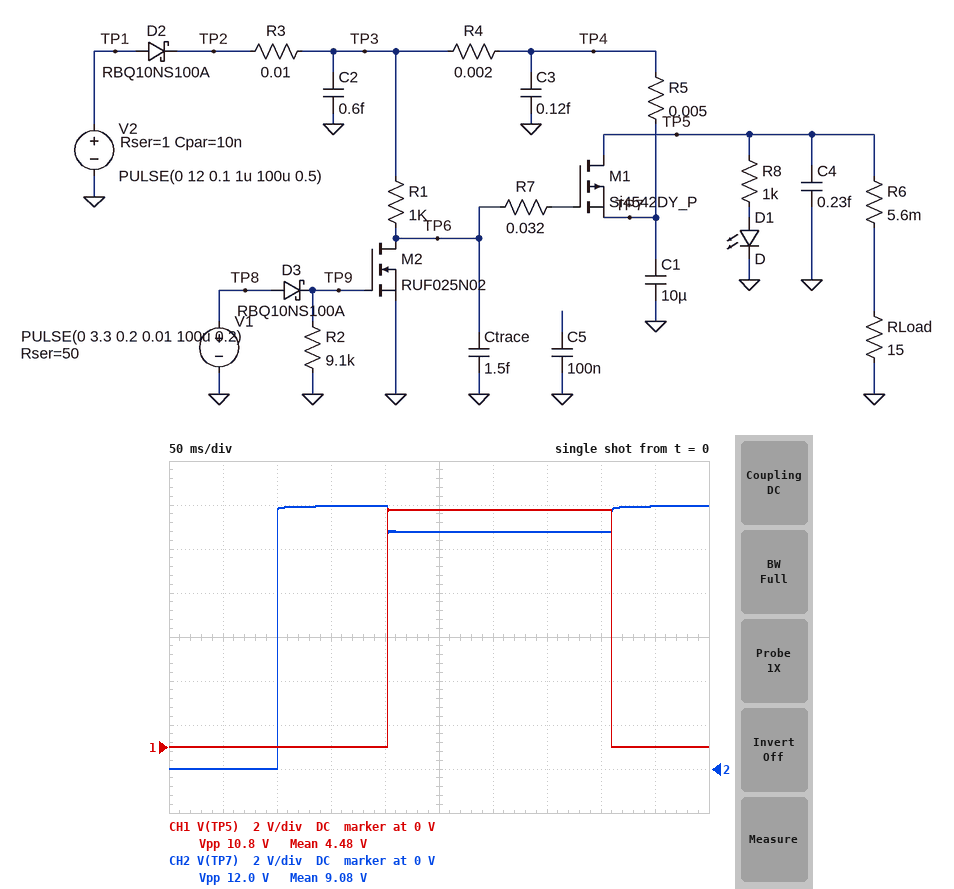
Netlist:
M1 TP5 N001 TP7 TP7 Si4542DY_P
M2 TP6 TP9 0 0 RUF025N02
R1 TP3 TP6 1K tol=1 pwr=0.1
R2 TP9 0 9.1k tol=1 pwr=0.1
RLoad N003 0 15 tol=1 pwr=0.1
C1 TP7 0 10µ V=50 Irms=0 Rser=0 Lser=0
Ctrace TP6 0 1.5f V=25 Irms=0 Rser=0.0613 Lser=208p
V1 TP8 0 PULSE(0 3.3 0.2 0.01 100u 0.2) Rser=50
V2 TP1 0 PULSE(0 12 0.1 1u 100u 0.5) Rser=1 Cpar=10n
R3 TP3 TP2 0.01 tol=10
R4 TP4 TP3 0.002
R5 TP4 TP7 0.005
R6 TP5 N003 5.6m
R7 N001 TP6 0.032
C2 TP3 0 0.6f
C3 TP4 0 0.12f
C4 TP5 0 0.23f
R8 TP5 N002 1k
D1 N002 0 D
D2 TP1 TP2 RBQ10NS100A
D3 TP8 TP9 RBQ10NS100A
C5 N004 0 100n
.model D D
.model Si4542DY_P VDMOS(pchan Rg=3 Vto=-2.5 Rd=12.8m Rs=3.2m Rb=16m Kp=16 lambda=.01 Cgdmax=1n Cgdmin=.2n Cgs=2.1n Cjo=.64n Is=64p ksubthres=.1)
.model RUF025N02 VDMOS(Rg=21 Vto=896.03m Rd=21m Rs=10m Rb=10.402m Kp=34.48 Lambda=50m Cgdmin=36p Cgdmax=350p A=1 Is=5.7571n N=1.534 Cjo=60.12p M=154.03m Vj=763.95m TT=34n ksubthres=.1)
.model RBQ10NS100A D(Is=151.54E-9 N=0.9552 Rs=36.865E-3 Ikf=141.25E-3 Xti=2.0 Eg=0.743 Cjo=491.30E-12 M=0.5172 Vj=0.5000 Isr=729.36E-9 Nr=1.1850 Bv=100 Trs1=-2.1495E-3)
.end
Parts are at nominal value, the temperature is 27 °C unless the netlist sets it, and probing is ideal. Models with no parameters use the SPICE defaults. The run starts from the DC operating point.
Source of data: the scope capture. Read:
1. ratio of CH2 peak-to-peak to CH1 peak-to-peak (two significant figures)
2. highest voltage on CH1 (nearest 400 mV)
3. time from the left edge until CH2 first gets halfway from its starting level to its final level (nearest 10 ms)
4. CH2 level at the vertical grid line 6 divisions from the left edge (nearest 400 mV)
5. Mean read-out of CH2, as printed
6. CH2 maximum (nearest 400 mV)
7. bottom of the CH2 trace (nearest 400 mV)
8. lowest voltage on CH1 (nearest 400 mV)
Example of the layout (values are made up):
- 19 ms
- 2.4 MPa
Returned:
- 1.1
- 10.8 V
- 100 ms
- 10.8 V
- 9.08 V
- 12.0 V
- 0 V
- 0 V
